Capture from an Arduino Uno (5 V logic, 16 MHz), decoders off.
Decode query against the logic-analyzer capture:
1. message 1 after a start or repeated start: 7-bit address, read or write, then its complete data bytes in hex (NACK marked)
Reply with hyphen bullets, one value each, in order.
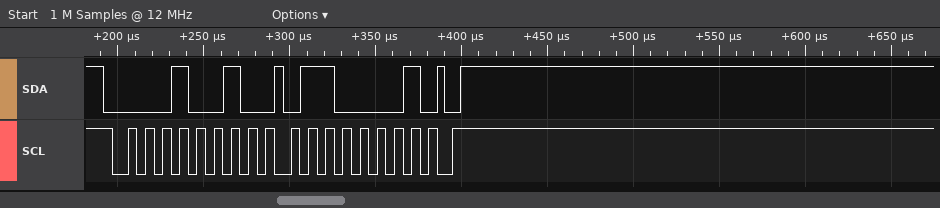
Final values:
- 0x09 write: 61
